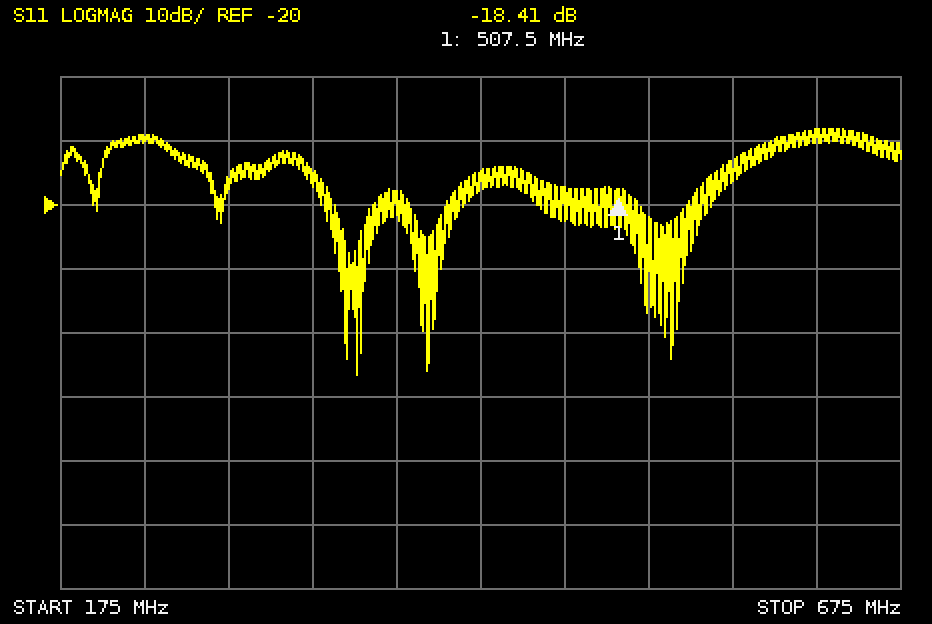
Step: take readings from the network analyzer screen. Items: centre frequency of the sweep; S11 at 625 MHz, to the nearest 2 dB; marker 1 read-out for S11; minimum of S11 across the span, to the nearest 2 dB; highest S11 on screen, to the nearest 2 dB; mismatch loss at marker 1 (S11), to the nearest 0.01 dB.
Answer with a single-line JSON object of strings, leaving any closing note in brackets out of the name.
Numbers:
{"centre frequency of the sweep": "425 MHz", "S11 at 625 MHz, to the nearest 2 dB": "-8 dB", "marker 1 read-out for S11": "-18.41 dB", "minimum of S11 across the span, to the nearest 2 dB": "-46 dB", "highest S11 on screen, to the nearest 2 dB": "-8 dB", "mismatch loss at marker 1 (S11), to the nearest 0.01 dB": "0.06 dB"}
